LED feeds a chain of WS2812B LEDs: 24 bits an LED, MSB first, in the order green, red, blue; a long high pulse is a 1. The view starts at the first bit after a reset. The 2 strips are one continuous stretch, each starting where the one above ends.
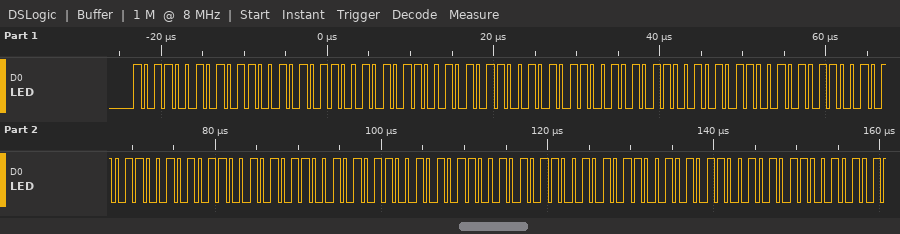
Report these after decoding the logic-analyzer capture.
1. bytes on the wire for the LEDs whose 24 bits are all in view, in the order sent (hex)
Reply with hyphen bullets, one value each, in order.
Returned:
- B2 B2 B2 B2 B2 B2 B2 B2 B2 B2 B2 B2 B2 B2 B2 B2 B2 B2
